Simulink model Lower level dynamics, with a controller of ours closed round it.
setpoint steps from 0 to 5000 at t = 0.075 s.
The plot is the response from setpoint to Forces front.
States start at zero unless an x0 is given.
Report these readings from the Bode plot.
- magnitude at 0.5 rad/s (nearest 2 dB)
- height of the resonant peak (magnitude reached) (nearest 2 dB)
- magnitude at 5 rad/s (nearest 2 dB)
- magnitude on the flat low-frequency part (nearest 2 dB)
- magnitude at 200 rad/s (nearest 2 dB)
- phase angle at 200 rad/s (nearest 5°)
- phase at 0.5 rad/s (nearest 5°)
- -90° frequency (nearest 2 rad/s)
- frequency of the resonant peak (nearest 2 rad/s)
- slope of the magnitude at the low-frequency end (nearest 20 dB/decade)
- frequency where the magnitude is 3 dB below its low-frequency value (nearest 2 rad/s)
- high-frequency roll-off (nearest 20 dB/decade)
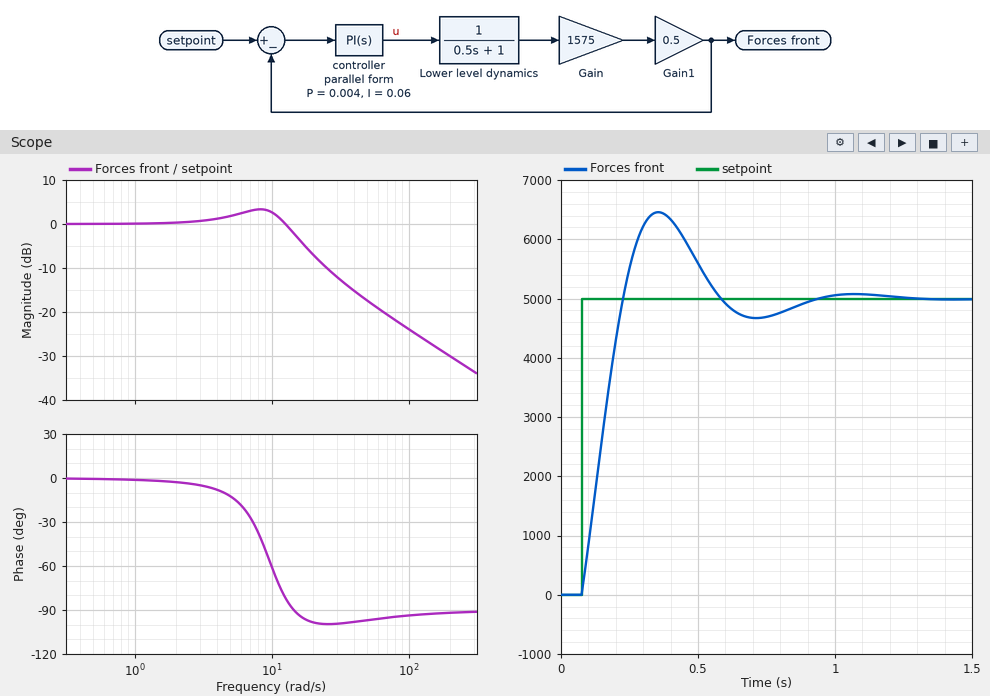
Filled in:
0 dB
4 dB
2 dB
0 dB
-30 dB
-90°
0°
14 rad/s
8 rad/s
0 dB/decade
16 rad/s
-20 dB/decade
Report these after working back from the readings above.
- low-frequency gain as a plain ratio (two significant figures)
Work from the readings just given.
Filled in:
1.0
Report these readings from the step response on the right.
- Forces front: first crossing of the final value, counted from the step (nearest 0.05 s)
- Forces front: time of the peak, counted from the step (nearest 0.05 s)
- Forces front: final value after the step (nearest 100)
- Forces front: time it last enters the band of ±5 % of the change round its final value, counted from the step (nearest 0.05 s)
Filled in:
0.15 s
0.30 s
5000
0.70 s
